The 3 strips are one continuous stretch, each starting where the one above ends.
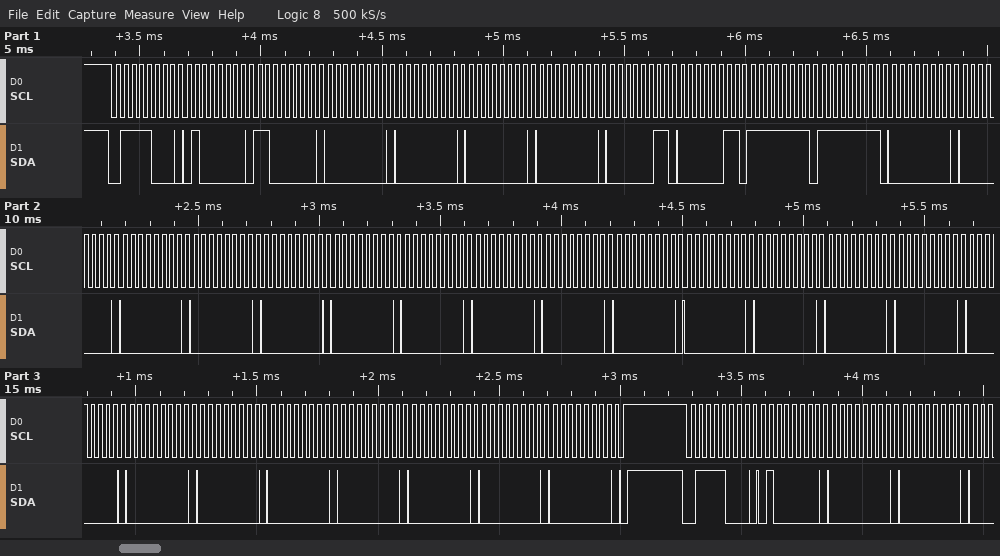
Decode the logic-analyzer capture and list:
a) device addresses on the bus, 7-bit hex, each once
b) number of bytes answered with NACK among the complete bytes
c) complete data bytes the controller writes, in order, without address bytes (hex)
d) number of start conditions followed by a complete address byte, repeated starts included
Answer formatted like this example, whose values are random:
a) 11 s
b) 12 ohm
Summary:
a) 0x3C
b) 0
c) 40 C0 00 00 00 00 03 03 FF FF 00 00 00 00 00 00 00 00 00 00 00 00 00 00 00 00 00 00 00 00 00 00 40 00 00
d) 2
